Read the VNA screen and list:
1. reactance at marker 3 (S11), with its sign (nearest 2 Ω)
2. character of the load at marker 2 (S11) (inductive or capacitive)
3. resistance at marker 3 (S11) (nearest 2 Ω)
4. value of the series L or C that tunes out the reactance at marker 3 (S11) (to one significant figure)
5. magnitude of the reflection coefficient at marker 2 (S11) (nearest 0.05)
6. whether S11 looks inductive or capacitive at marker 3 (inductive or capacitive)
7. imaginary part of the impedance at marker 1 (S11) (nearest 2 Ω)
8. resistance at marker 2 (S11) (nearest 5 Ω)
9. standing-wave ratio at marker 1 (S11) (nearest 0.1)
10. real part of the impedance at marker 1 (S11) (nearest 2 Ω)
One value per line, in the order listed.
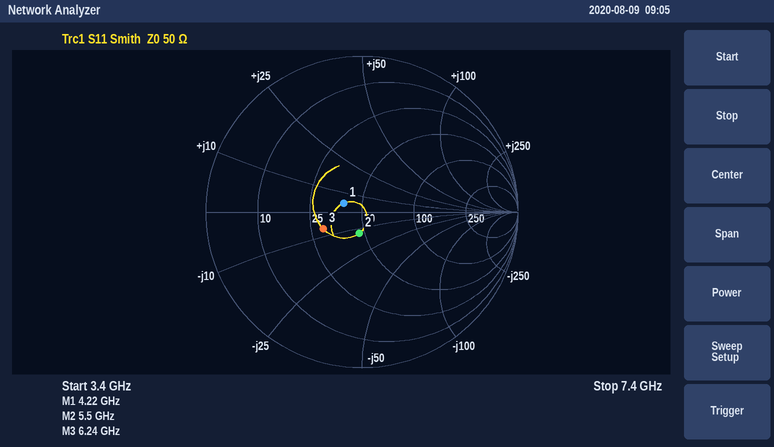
-6 Ω
capacitive
30 Ω
200 pH
0.15
capacitive
+4 Ω
45 Ω
1.3
40 Ω
